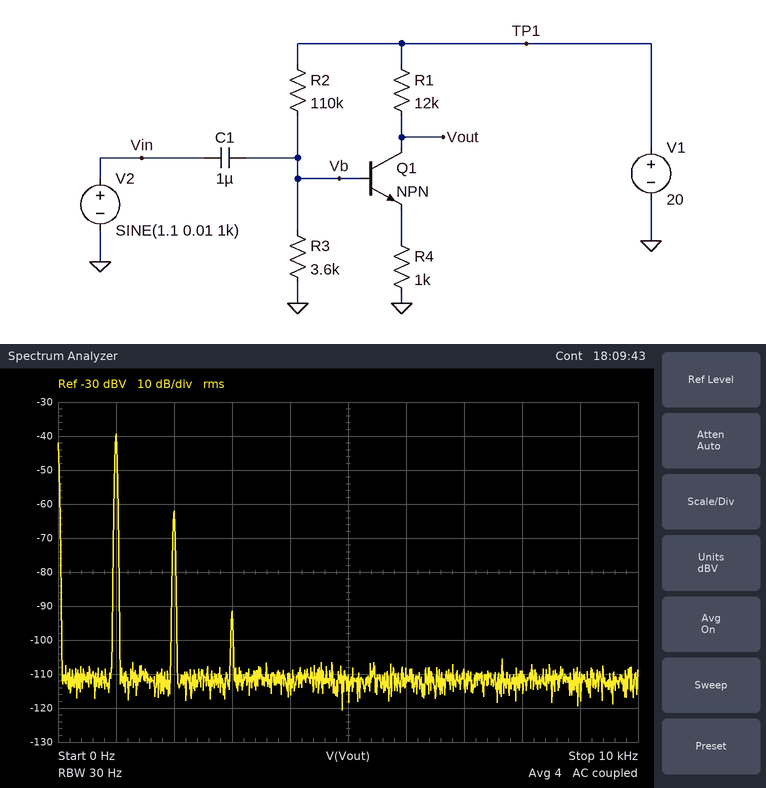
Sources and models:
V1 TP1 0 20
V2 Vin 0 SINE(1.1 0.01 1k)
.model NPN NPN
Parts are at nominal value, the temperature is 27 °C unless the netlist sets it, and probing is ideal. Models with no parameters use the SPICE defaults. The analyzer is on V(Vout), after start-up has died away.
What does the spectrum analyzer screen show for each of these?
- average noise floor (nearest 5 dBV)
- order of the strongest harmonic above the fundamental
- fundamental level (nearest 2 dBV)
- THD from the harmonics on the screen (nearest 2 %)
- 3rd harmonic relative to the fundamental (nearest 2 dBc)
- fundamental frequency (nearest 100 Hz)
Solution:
-110 dBV
2
-40 dBV
8 %
-52 dBc
1.0 kHz
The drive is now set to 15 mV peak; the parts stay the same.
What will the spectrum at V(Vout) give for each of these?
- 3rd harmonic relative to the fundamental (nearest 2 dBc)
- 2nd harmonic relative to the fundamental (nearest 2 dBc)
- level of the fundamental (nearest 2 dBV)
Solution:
-46 dBc
-20 dBc
-36 dBV
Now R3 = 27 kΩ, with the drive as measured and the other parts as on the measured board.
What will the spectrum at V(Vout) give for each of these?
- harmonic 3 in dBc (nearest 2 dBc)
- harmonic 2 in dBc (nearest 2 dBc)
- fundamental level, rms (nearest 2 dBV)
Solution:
-54 dBc
-28 dBc
-48 dBV
